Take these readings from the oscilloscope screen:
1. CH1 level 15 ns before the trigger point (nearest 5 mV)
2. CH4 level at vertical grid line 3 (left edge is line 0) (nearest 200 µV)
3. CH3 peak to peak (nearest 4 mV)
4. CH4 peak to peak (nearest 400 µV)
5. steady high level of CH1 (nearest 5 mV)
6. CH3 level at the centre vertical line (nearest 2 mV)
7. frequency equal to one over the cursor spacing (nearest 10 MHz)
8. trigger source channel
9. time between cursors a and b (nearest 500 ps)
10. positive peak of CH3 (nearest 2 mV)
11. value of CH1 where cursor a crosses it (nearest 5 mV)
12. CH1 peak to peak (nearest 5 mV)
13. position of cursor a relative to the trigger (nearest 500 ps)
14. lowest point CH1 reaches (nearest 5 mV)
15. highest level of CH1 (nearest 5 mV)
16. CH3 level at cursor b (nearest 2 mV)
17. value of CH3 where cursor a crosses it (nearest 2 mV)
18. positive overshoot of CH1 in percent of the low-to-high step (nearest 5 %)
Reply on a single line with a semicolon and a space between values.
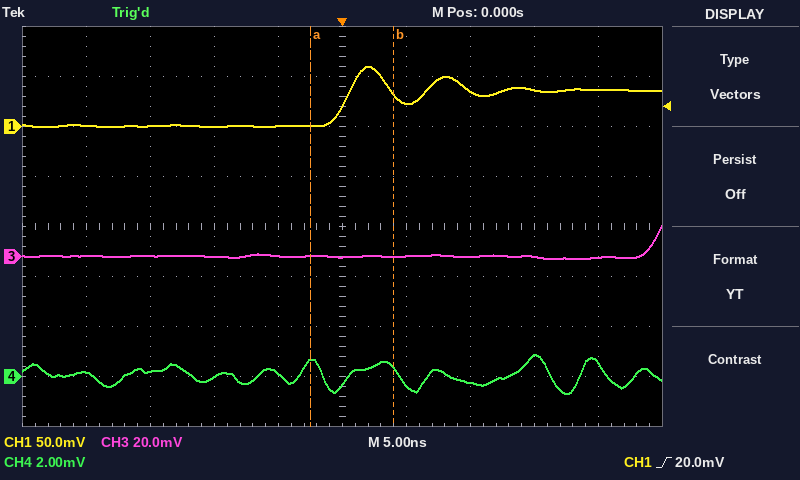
0 mV; 0.0 mV; 12 mV; 1.6 mV; 35 mV; 0 mV; 150 MHz; CH1; 6.5 ns; 12 mV; 0 mV; 60 mV; -2.5 ns; 0 mV; 60 mV; 0 mV; 0 mV; 65 %
